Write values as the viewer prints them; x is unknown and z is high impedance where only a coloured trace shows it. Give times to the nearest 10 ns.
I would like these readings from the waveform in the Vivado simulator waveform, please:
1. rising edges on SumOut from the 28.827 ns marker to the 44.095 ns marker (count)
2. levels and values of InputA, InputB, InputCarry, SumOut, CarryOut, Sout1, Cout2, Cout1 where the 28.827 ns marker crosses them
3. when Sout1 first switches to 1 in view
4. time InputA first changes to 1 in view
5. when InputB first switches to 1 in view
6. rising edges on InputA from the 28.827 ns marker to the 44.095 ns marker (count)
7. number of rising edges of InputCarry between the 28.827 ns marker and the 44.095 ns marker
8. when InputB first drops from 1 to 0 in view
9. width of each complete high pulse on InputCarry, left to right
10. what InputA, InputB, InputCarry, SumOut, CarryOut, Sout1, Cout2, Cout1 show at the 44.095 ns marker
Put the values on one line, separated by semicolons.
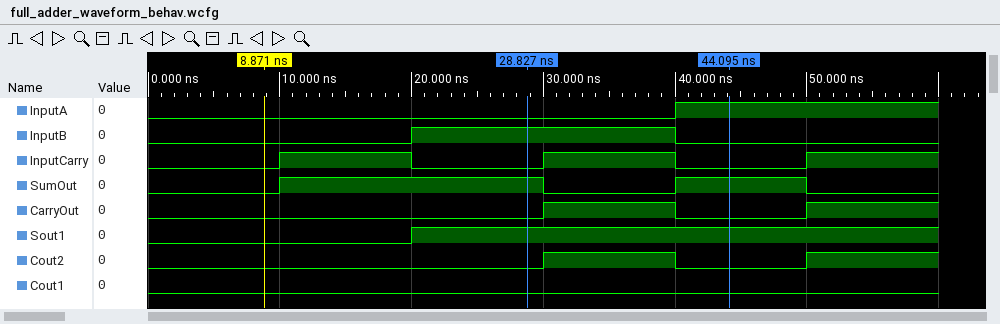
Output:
1; InputA=0, InputB=1, InputCarry=0, SumOut=1, CarryOut=0, Sout1=1, Cout2=0, Cout1=0; 20 ns; 40 ns; 20 ns; 1; 1; 40 ns; 10 ns, 10 ns; InputA=1, InputB=0, InputCarry=0, SumOut=1, CarryOut=0, Sout1=1, Cout2=0, Cout1=0
